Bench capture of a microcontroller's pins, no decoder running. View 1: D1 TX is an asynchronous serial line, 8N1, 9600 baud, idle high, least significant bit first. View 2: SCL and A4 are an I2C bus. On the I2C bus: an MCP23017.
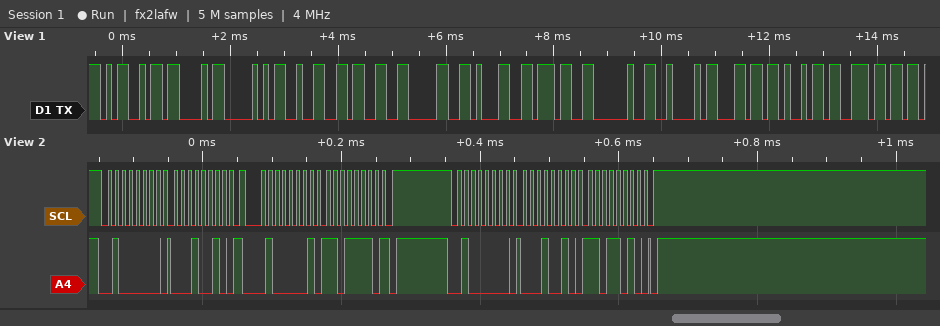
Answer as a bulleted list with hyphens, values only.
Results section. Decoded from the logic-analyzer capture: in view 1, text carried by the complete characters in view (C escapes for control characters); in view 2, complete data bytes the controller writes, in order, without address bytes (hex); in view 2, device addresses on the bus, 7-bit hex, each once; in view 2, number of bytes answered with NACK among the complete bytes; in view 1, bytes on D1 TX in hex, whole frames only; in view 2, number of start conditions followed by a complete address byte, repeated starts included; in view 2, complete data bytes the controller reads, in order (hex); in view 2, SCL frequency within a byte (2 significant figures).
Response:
- "MCP23017 Blin"
- 12 12 DA
- 0x20
- 1
- 4D 43 50 32 33 30 31 37 20 42 6C 69 6E
- 3
- DE
- 100 kHz
